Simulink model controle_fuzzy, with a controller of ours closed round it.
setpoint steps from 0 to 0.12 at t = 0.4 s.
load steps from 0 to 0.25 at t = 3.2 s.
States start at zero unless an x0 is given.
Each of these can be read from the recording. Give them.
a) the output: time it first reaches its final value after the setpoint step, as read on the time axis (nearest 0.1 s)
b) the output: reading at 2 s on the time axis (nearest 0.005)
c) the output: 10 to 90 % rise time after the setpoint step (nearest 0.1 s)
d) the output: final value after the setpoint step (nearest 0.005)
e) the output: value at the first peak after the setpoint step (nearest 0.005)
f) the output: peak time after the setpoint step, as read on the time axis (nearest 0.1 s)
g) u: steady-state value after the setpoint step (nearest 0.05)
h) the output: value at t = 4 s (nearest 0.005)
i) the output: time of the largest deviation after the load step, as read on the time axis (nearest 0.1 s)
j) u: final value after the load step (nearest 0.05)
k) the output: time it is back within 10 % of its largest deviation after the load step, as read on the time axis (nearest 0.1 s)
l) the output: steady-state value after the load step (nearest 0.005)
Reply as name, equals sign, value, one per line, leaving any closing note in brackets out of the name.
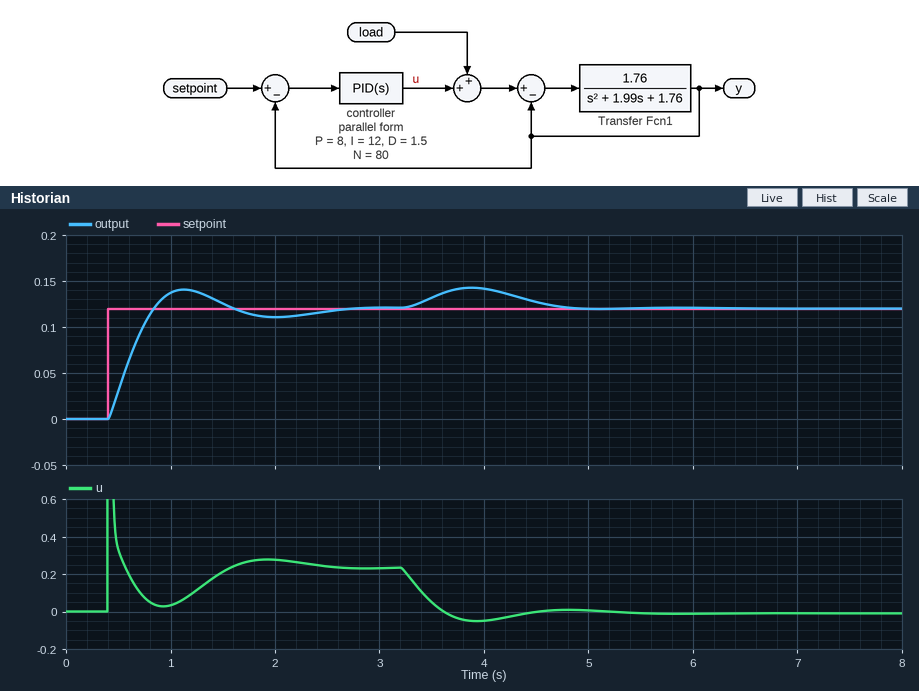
the output: time it first reaches its final value after the setpoint step, as read on the time axis = 0.8 s
the output: reading at 2 s on the time axis = 0.110
the output: 10 to 90 % rise time after the setpoint step = 0.3 s
the output: final value after the setpoint step = 0.120
the output: value at the first peak after the setpoint step = 0.140
the output: peak time after the setpoint step, as read on the time axis = 1.1 s
u: steady-state value after the setpoint step = 0.25
the output: value at t = 4 s = 0.140
the output: time of the largest deviation after the load step, as read on the time axis = 3.9 s
u: final value after the load step = 0.00
the output: time it is back within 10 % of its largest deviation after the load step, as read on the time axis = 4.7 s
the output: steady-state value after the load step = 0.120
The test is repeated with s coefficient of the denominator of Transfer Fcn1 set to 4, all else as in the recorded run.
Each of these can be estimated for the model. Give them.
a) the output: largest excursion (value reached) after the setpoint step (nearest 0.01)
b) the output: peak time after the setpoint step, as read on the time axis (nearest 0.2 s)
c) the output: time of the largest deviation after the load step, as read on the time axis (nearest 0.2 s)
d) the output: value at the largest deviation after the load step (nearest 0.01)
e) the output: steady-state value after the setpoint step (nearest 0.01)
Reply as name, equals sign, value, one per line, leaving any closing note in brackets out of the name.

the output: largest excursion (value reached) after the setpoint step = 0.13
the output: peak time after the setpoint step, as read on the time axis = 1.4 s
the output: time of the largest deviation after the load step, as read on the time axis = 4.0 s
the output: value at the largest deviation after the load step = 0.14
the output: steady-state value after the setpoint step = 0.12
